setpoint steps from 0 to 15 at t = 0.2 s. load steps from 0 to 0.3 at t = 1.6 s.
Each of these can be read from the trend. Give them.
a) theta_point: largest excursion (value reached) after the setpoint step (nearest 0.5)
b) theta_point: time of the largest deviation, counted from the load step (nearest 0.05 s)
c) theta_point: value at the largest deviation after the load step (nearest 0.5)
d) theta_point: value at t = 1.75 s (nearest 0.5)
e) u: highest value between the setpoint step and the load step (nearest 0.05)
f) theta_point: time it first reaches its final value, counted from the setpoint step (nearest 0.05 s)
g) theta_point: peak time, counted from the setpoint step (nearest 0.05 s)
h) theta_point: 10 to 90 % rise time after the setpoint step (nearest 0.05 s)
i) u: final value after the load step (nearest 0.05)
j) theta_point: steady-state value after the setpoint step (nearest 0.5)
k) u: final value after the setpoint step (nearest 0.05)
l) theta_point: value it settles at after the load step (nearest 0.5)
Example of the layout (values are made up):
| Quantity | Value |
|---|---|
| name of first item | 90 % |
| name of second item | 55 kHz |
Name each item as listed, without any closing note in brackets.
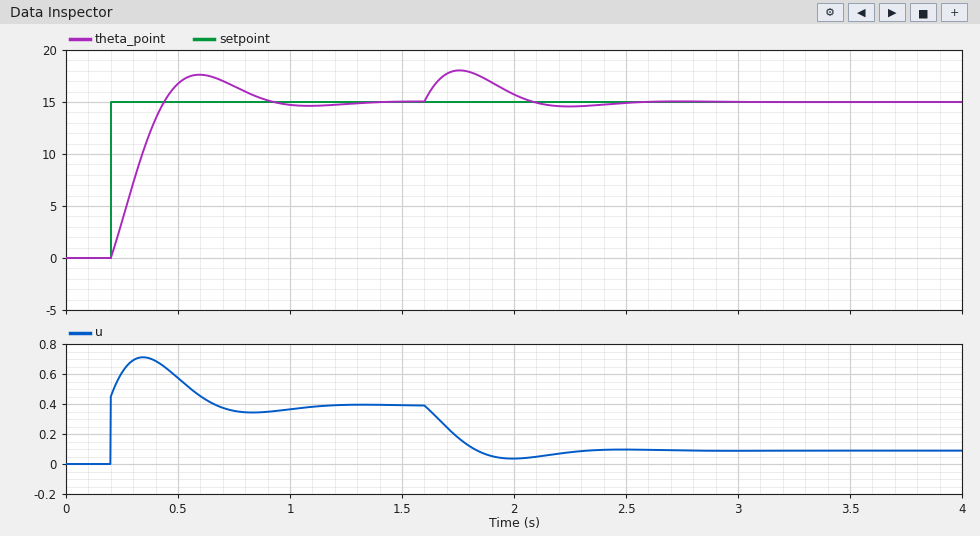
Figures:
| Quantity | Value |
|---|---|
| theta_point: largest excursion (value reached) after the setpoint step | 17.5 |
| theta_point: time of the largest deviation, counted from the load step | 0.15 s |
| theta_point: value at the largest deviation after the load step | 18.0 |
| theta_point: value at t = 1.75 s | 18.0 |
| u: highest value between the setpoint step and the load step | 0.70 |
| theta_point: time it first reaches its final value, counted from the setpoint step | 0.25 s |
| theta_point: peak time, counted from the setpoint step | 0.40 s |
| theta_point: 10 to 90 % rise time after the setpoint step | 0.20 s |
| u: final value after the load step | 0.10 |
| theta_point: steady-state value after the setpoint step | 15.0 |
| u: final value after the setpoint step | 0.40 |
| theta_point: value it settles at after the load step | 15.0 |
